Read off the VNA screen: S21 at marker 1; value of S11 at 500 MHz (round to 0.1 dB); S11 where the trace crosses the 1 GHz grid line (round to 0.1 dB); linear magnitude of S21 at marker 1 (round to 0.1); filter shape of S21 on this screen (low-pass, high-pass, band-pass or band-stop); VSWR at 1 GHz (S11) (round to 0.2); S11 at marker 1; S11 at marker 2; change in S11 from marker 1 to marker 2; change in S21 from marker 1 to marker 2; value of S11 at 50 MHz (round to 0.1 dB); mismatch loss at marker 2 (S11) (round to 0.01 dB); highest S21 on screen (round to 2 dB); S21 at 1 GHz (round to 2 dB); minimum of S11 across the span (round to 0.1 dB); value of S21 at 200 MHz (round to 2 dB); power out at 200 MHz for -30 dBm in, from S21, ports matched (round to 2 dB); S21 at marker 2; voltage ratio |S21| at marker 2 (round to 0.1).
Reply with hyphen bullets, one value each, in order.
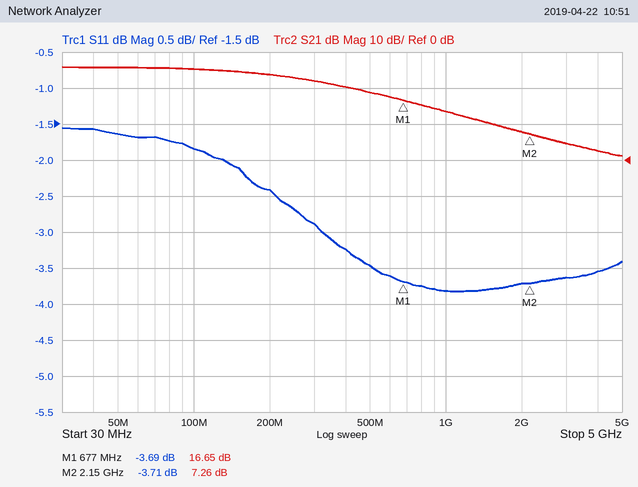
- 16.65 dB
- -3.5 dB
- -3.8 dB
- 6.8
- low-pass
- 4.6
- -3.69 dB
- -3.71 dB
- -0.02 dB
- -9.39 dB
- -1.6 dB
- 2.41 dB
- 26 dB
- 14 dB
- -3.8 dB
- 24 dB
- -6 dBm
- 7.26 dB
- 2.3
